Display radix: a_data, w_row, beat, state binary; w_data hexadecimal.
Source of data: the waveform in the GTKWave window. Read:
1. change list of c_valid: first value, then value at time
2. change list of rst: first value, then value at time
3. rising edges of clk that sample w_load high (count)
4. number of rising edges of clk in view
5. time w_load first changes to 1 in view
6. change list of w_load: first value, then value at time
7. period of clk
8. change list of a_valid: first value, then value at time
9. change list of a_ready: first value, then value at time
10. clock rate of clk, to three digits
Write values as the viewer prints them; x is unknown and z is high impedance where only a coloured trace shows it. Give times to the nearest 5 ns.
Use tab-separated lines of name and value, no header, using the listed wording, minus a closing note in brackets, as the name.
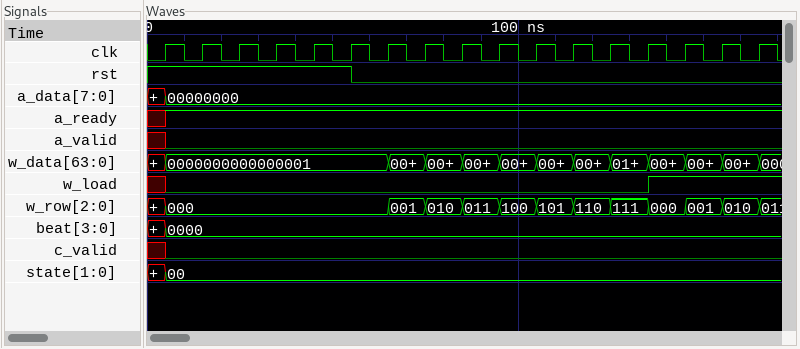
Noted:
change list of c_valid: first value, then value at time	x, 0 at 5 ns
change list of rst: first value, then value at time	1, 0 at 55 ns
rising edges of clk that sample w_load high	3
number of rising edges of clk in view	17
time w_load first changes to 1 in view	135 ns
change list of w_load: first value, then value at time	x, 0 at 5 ns, 1 at 135 ns
period of clk	10 ns
change list of a_valid: first value, then value at time	x, 0 at 5 ns
change list of a_ready: first value, then value at time	x, 1 at 5 ns
clock rate of clk, to three digits	100 MHz
